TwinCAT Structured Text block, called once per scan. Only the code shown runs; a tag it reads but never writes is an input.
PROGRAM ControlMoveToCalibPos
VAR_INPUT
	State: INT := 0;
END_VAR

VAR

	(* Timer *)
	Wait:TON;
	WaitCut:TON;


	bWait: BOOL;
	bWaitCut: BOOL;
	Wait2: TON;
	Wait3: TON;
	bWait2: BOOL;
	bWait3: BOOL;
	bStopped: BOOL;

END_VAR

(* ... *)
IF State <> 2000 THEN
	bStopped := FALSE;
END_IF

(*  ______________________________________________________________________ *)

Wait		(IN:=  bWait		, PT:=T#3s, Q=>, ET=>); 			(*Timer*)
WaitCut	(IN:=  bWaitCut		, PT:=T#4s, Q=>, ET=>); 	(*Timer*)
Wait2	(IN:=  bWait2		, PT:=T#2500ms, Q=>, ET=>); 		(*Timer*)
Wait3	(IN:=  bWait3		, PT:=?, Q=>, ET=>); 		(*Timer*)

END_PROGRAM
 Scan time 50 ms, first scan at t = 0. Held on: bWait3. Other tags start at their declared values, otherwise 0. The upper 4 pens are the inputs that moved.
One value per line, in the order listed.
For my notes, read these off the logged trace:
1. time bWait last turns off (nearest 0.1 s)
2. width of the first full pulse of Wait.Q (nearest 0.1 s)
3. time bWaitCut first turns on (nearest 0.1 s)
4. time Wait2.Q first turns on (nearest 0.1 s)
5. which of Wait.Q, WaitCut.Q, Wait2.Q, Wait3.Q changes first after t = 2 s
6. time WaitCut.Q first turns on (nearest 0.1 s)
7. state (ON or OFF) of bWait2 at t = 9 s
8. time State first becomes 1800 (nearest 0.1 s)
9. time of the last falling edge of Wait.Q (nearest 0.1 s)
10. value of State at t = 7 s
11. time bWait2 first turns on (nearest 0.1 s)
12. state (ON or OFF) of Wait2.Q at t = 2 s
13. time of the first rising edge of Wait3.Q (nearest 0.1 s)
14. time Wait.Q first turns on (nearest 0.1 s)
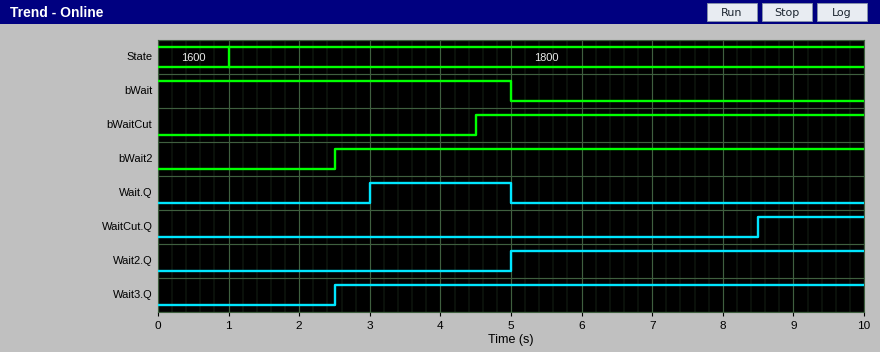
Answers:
5.0 s
2.0 s
4.5 s
5.0 s
Wait3.Q
8.5 s
ON
1.0 s
5.0 s
1800
2.5 s
OFF
2.5 s
3.0 s
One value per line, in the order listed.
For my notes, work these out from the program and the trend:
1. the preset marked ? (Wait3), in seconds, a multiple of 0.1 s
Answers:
2.5 s
